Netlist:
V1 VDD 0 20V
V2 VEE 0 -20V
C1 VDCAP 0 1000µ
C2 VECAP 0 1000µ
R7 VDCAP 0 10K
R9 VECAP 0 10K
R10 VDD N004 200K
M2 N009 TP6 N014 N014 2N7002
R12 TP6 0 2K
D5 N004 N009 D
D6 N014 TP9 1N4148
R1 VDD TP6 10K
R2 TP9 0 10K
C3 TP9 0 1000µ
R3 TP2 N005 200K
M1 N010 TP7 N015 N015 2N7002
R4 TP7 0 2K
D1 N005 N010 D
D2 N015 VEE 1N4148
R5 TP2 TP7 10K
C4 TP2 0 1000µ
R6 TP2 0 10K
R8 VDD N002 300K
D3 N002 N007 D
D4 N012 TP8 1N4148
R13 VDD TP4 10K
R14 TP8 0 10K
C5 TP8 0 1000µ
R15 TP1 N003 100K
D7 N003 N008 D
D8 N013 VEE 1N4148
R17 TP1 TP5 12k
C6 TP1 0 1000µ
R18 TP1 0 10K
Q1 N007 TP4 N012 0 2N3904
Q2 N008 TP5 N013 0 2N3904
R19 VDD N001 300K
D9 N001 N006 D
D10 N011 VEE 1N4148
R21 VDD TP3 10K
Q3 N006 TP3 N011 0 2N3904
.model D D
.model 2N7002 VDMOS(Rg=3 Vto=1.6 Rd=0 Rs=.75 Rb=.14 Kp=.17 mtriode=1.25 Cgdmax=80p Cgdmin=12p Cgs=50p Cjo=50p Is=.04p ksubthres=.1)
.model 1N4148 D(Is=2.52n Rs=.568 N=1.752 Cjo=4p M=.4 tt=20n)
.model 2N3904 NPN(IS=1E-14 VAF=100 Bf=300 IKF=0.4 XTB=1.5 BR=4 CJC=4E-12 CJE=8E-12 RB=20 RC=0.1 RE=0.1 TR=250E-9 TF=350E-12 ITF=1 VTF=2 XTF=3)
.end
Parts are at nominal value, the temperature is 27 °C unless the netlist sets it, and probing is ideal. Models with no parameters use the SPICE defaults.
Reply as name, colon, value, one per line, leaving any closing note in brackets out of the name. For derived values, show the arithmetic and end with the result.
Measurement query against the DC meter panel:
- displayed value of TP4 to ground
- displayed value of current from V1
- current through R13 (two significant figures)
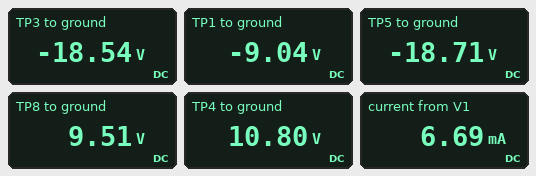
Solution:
displayed value of TP4 to ground: 10.80 V
displayed value of current from V1: 6.69 mA
current through R13: (20 V - 10.8 V) / 10 kΩ = 920 µA
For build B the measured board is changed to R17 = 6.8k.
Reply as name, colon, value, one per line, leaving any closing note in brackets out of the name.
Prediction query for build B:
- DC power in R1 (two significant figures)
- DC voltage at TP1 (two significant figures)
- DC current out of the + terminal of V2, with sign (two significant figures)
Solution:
DC power in R1: 28 mW
DC voltage at TP1: -11 V
DC current out of the + terminal of V2, with sign: -5.2 mA
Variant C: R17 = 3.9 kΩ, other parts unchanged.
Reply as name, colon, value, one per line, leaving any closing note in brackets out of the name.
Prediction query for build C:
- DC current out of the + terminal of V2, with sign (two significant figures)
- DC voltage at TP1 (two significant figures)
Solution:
DC current out of the + terminal of V2, with sign: -5.4 mA
DC voltage at TP1: -14 V
